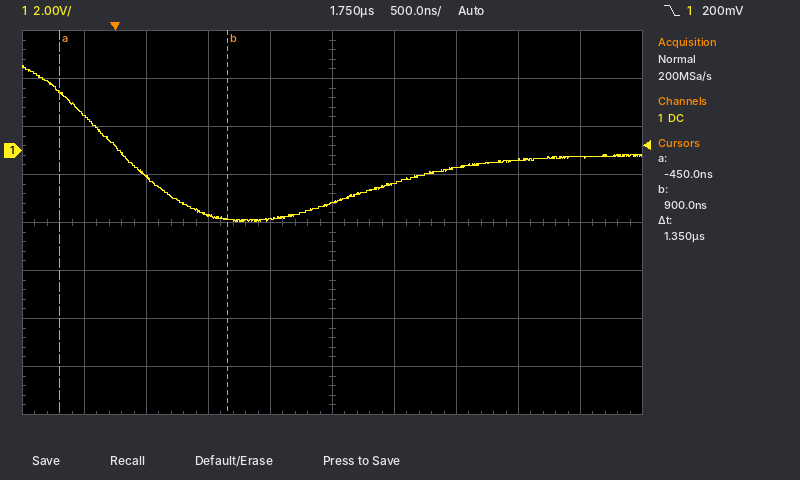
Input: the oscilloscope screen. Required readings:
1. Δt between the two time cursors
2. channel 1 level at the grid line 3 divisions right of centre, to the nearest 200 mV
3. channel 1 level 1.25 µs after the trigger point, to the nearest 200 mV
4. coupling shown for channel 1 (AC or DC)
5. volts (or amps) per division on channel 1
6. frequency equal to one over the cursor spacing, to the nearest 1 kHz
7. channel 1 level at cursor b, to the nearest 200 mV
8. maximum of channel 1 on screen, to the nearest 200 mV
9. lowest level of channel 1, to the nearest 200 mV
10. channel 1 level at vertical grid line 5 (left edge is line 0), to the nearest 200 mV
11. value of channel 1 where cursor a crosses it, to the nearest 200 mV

1.35 µs
-400 mV
-2.8 V
DC
2 V
741 kHz
-2.8 V
3.6 V
-3.0 V
-2.2 V
2.4 V
